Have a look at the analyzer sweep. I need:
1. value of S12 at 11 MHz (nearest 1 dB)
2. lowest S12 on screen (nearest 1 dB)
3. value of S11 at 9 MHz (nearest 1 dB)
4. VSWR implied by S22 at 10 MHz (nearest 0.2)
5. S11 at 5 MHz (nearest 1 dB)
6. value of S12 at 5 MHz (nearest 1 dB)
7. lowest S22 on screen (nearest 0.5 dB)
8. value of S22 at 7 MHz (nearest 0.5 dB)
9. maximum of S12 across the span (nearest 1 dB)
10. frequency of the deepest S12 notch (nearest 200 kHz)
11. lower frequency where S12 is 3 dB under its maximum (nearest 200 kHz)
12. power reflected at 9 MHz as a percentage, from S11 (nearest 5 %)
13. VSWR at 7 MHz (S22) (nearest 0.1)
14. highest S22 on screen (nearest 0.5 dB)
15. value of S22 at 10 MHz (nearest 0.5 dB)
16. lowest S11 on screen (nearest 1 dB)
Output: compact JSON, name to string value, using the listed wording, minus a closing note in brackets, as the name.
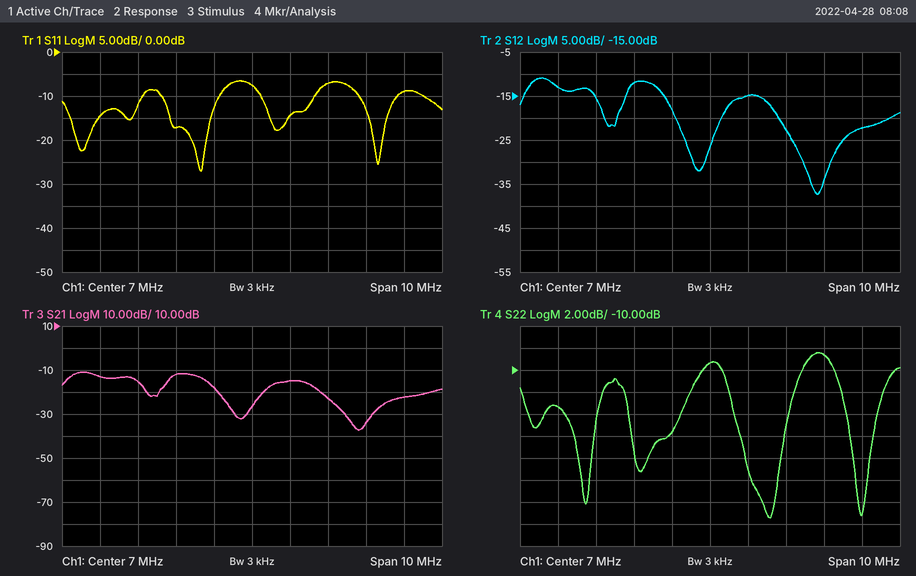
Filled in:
{"value of S12 at 11 MHz": "-22 dB", "lowest S12 on screen": "-37 dB", "value of S11 at 9 MHz": "-7 dB", "VSWR implied by S22 at 10 MHz": "2.2", "S11 at 5 MHz": "-17 dB", "value of S12 at 5 MHz": "-12 dB", "lowest S22 on screen": "-23.5 dB", "value of S22 at 7 MHz": "-9.5 dB", "maximum of S12 across the span": "-11 dB", "frequency of the deepest S12 notch": "9.8 MHz", "lower frequency where S12 is 3 dB under its maximum": "2.2 MHz", "power reflected at 9 MHz as a percentage, from S11": "20 %", "VSWR at 7 MHz (S22)": "2.0", "highest S22 on screen": "-8.5 dB", "value of S22 at 10 MHz": "-8.5 dB", "lowest S11 on screen": "-27 dB"}
